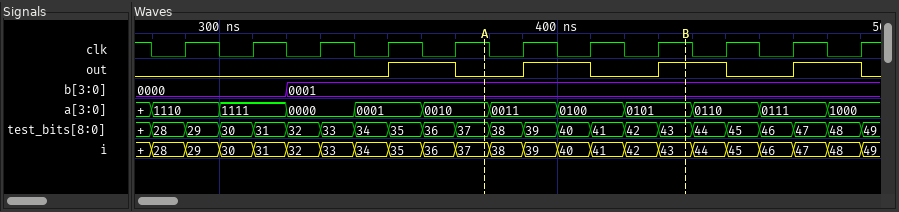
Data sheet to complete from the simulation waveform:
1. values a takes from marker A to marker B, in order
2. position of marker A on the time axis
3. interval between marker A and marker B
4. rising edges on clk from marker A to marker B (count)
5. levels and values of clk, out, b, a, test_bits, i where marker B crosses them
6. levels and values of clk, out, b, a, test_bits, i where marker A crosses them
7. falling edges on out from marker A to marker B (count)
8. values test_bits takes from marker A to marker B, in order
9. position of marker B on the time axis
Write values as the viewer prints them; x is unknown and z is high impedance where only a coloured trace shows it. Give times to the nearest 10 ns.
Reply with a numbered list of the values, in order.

1. 0010, 0011, 0100, 0101
2. 380 ns
3. 60 ns
4. 3
5. clk=1, out=1, b=0001, a=0101, test_bits=43, i=43
6. clk=1, out=0, b=0001, a=0010, test_bits=37, i=37
7. 1
8. 37, 38, 39, 40, 41, 42, 43
9. 440 ns
